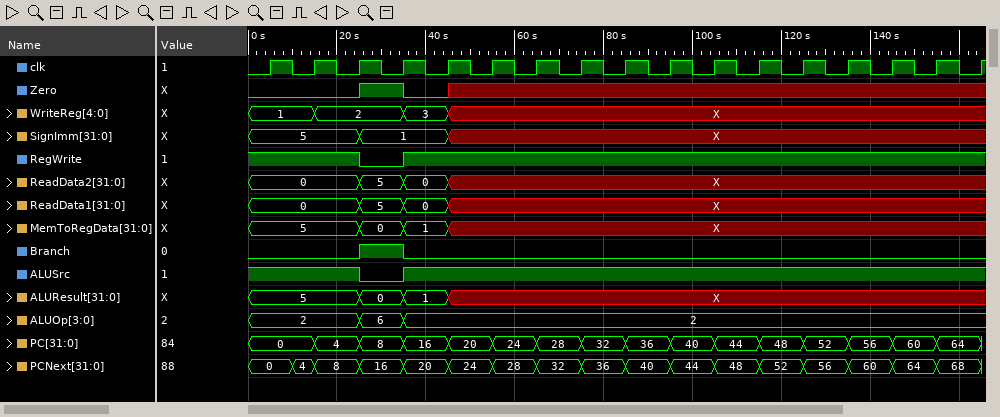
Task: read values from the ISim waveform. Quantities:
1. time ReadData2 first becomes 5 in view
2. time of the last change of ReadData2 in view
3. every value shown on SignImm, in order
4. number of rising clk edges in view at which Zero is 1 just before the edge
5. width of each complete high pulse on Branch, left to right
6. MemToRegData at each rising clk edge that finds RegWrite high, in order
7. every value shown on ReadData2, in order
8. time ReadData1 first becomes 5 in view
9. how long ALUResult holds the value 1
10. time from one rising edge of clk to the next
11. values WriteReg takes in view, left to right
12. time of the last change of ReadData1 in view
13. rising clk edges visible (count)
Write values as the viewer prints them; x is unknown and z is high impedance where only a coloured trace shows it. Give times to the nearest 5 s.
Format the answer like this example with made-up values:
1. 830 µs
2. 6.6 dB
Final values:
1. 25 s
2. 45 s
3. 5, 1, X
4. 1
5. 10 s
6. 5, 5, 5, 1, X, X, X, X, X, X, X, X, X, X, X, X
7. 0, 5, 0, X
8. 25 s
9. 10 s
10. 10 s
11. 1, 2, 3, X
12. 45 s
13. 17
